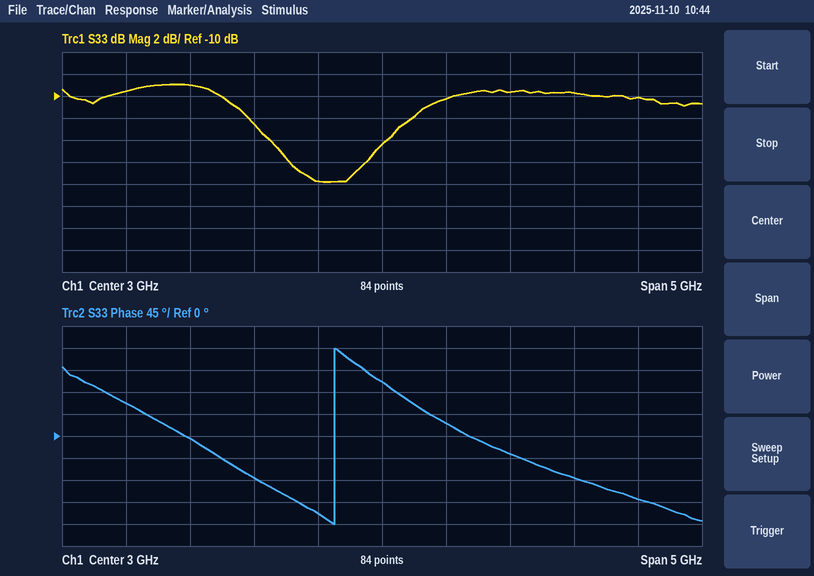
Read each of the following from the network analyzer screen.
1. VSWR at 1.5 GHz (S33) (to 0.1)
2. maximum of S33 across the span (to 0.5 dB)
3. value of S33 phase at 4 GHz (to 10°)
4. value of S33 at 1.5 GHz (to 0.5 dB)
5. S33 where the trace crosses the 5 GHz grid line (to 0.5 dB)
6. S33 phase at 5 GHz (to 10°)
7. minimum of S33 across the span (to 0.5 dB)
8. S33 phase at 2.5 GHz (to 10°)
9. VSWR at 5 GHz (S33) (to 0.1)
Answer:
2.1
-9.0 dB
-40°
-9.0 dB
-10.0 dB
-130°
-18.0 dB
-160°
1.9
